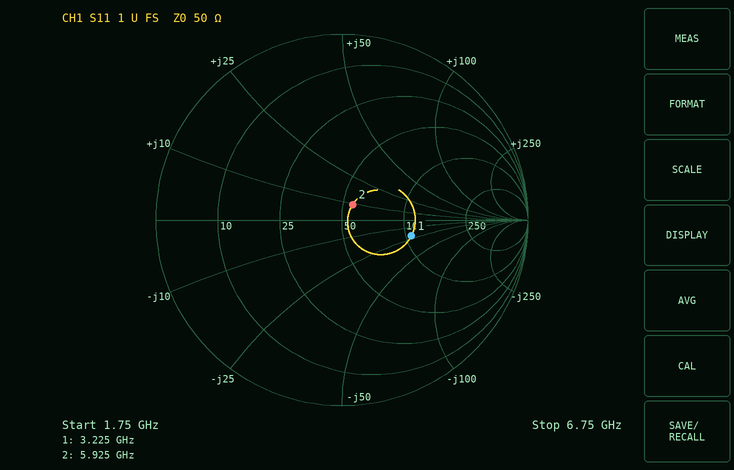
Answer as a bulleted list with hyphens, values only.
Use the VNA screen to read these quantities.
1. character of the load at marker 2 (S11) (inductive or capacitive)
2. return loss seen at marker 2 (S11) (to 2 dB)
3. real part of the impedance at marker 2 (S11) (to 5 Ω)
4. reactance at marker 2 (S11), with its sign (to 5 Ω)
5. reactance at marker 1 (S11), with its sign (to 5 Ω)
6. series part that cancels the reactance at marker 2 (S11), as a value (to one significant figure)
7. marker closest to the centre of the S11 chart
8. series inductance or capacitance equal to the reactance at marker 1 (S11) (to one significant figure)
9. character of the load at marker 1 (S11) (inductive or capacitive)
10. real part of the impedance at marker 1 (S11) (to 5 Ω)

- inductive
- 20 dB
- 55 Ω
- +10 Ω
- -20 Ω
- 3 pF
- marker 2
- 2 pF
- capacitive
- 105 Ω
